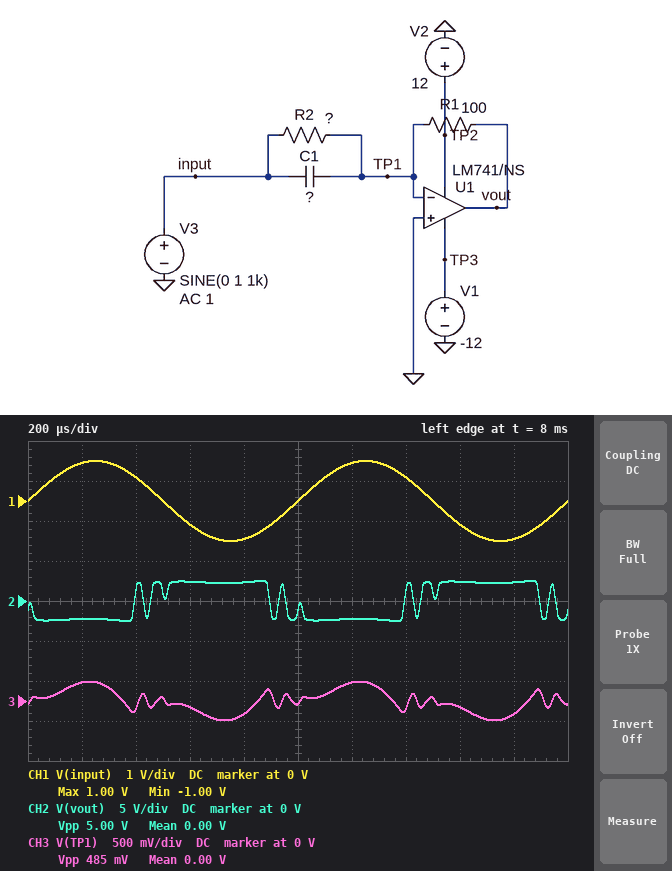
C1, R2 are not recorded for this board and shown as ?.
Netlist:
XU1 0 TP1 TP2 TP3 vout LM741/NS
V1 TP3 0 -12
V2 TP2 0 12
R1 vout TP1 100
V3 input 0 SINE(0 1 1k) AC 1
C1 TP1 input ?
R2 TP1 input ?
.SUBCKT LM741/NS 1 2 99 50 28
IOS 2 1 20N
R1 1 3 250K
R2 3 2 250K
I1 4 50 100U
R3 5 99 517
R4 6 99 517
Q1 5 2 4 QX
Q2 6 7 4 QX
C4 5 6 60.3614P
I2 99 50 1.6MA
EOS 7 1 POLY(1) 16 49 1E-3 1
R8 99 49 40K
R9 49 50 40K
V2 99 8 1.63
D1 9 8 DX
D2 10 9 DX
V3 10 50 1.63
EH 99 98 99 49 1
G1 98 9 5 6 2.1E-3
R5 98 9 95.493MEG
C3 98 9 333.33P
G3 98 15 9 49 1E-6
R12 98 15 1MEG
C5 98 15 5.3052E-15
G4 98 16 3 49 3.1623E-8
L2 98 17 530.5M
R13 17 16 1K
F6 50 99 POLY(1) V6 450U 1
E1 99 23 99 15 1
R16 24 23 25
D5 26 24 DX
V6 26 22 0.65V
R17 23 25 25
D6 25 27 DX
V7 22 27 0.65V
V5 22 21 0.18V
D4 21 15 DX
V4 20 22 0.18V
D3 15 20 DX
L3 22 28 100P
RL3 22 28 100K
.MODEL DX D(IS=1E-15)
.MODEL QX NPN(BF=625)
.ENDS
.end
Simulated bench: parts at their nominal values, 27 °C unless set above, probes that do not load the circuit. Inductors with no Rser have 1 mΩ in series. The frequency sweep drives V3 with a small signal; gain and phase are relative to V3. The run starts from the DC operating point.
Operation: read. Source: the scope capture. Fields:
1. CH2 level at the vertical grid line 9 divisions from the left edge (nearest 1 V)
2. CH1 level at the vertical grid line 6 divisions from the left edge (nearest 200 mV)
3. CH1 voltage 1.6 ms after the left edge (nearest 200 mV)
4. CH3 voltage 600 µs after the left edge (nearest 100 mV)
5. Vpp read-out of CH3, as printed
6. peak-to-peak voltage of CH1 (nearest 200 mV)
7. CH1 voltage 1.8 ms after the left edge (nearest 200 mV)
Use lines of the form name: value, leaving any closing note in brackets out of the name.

CH2 level at the vertical grid line 9 divisions from the left edge: 2 V
CH1 level at the vertical grid line 6 divisions from the left edge: 1.0 V
CH1 voltage 1.6 ms after the left edge: -600 mV
CH3 voltage 600 µs after the left edge: -100 mV
Vpp read-out of CH3, as printed: 485 mV
peak-to-peak voltage of CH1: 2.0 V
CH1 voltage 1.8 ms after the left edge: -1.0 V
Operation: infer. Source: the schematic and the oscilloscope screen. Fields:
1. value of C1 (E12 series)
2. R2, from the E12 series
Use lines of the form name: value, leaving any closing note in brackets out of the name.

value of C1: 2.7 µF
R2, from the E12 series: 33 Ω
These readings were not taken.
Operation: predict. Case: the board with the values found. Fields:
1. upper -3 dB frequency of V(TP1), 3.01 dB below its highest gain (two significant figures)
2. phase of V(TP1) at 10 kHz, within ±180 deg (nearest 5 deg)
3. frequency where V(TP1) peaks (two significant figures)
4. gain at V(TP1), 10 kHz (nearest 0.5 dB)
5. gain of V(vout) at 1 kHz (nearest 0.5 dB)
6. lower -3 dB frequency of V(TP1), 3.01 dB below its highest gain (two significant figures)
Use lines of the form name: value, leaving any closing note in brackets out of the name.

upper -3 dB frequency of V(TP1), 3.01 dB below its highest gain: 16 kHz
phase of V(TP1) at 10 kHz, within ±180 deg: 160 deg
frequency where V(TP1) peaks: 15 kHz
gain at V(TP1), 10 kHz: -1.0 dB
gain of V(vout) at 1 kHz: 11.0 dB
lower -3 dB frequency of V(TP1), 3.01 dB below its highest gain: 14 kHz
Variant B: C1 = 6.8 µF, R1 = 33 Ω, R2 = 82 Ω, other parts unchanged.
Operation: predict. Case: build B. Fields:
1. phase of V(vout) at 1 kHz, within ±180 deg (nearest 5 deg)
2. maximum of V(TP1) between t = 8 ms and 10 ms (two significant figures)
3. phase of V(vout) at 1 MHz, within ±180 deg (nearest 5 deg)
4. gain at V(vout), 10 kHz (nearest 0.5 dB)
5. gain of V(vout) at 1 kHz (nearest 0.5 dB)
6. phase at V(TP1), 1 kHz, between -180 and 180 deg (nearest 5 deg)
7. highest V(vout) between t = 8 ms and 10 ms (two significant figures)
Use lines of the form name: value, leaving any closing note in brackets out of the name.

phase of V(vout) at 1 kHz, within ±180 deg: -105 deg
maximum of V(TP1) between t = 8 ms and 10 ms: 610 mV
phase of V(vout) at 1 MHz, within ±180 deg: 10 deg
gain at V(vout), 10 kHz: 44.0 dB
gain of V(vout) at 1 kHz: 3.5 dB
phase at V(TP1), 1 kHz, between -180 and 180 deg: 165 deg
highest V(vout) between t = 8 ms and 10 ms: 960 mV
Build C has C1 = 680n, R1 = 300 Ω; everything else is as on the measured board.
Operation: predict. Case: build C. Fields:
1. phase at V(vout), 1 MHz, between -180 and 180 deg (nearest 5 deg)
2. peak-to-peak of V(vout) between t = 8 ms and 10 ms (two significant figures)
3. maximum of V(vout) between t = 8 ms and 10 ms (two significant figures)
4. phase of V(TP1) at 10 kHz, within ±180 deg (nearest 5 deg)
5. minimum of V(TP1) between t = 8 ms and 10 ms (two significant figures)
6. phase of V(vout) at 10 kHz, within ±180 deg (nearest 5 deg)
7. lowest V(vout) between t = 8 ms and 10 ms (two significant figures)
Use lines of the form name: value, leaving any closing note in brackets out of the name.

phase at V(vout), 1 MHz, between -180 and 180 deg: 40 deg
peak-to-peak of V(vout) between t = 8 ms and 10 ms: 14 V
maximum of V(vout) between t = 8 ms and 10 ms: 7.2 V
phase of V(TP1) at 10 kHz, within ±180 deg: 135 deg
minimum of V(TP1) between t = 8 ms and 10 ms: -210 mV
phase of V(vout) at 10 kHz, within ±180 deg: -135 deg
lowest V(vout) between t = 8 ms and 10 ms: -7.2 V
